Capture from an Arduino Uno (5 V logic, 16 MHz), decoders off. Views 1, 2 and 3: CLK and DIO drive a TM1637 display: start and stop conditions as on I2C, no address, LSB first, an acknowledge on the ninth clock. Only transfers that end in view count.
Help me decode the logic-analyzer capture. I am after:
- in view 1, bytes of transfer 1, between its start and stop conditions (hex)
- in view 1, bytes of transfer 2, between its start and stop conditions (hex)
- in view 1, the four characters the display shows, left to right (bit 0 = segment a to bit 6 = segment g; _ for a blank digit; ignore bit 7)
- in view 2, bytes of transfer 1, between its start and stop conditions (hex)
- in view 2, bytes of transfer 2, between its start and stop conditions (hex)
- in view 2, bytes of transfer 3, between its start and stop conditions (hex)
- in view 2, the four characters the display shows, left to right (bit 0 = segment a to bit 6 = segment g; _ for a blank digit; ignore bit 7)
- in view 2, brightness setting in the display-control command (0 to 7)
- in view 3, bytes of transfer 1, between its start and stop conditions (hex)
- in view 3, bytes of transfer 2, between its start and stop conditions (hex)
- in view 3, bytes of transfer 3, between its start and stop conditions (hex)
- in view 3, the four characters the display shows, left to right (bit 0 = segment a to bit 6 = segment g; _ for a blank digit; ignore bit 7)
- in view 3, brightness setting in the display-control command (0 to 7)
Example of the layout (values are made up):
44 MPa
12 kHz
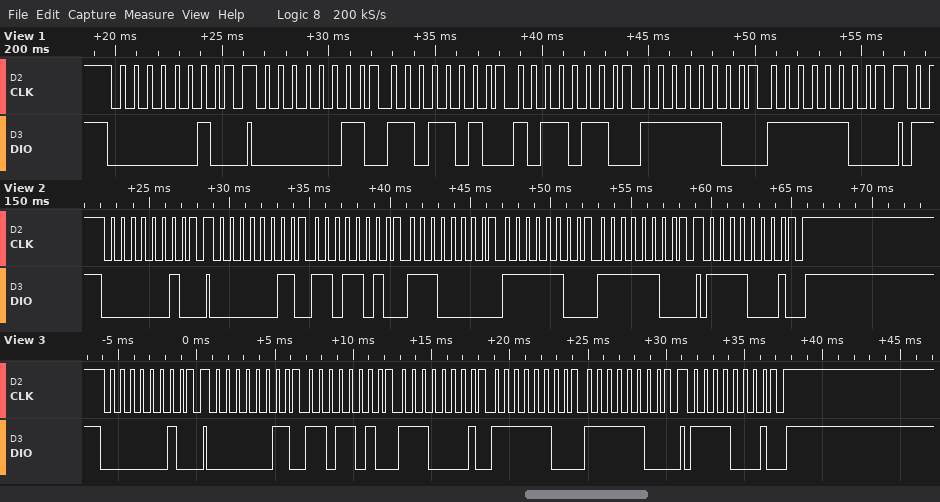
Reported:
40
C0 5B 6D 3F 3F
2500
40
C0 5B 07 3F 3F
8F
2700
7
40
C0 5B 87 3F 3F
8F
2700
7
